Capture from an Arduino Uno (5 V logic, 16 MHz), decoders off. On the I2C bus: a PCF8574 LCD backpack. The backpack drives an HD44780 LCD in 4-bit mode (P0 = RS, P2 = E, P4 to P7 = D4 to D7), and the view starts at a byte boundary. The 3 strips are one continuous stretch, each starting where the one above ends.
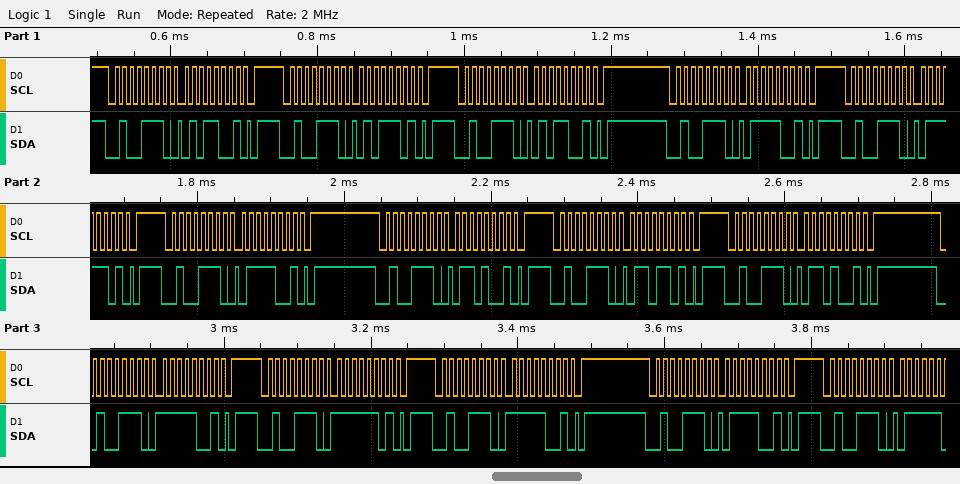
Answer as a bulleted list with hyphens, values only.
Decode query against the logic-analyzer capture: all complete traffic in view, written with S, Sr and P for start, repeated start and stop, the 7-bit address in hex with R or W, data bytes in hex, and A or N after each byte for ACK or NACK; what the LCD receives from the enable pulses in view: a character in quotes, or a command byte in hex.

- S 27W A 59 A P S 27W A 5D A P S 27W A 59 A P S 27W A 79 A P S 27W A 7D A P S 27W A 79 A P S 27W A 69 A P S 27W A 6D A P S 27W A 69 A P S 27W A F9 A P S 27W A FD A P S 27W A F9 A P S 27W A 79 A P S 27W A
- 'W' 'o'
